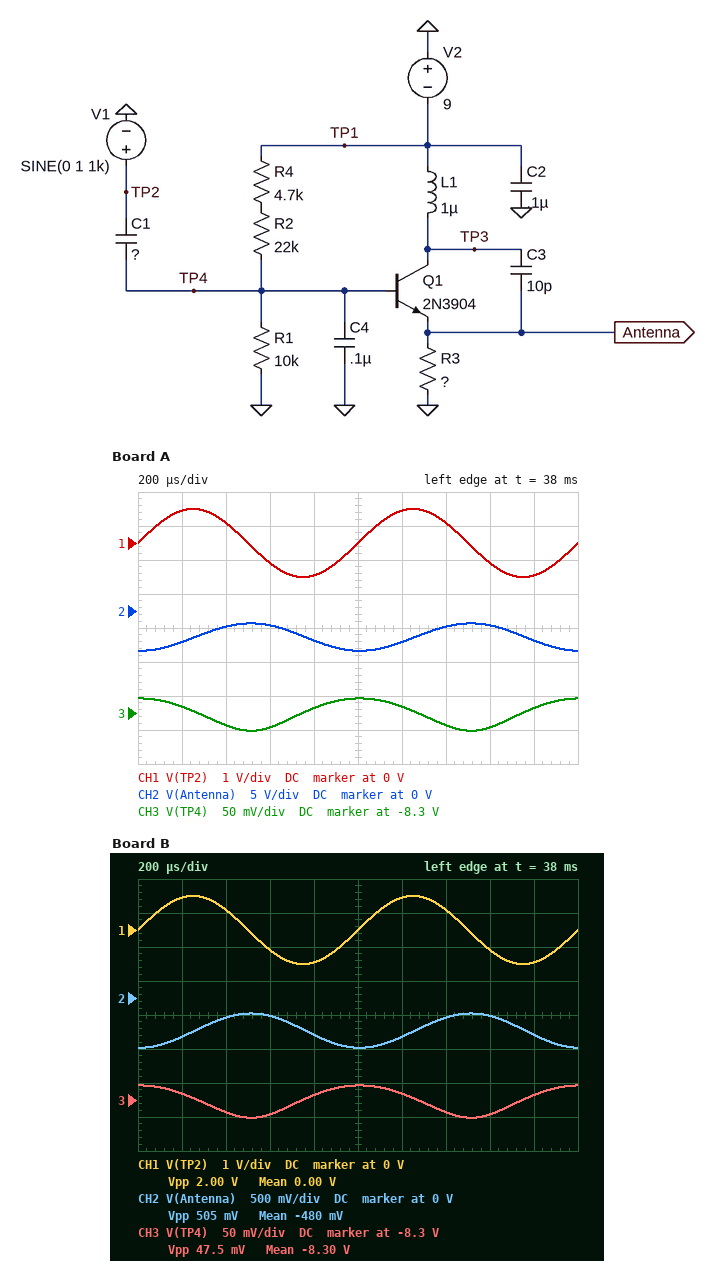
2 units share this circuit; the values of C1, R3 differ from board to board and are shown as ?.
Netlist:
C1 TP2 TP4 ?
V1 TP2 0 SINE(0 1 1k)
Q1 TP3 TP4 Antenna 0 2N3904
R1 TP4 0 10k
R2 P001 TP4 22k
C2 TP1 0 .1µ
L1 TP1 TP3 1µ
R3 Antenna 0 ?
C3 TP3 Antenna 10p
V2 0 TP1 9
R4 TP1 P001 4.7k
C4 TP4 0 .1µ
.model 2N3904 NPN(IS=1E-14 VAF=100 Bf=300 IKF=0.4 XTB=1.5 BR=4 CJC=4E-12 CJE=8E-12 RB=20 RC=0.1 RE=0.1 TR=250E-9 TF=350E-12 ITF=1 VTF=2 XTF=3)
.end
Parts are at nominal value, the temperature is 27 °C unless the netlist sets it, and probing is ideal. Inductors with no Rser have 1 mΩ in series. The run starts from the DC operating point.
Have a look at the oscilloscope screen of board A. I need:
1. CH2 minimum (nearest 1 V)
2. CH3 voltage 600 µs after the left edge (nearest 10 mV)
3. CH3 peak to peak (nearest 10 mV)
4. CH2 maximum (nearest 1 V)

-6 V
-8.32 V
50 mV
-2 V
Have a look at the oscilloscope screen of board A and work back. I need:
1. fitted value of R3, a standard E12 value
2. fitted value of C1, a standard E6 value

1.2 kΩ
68 nF
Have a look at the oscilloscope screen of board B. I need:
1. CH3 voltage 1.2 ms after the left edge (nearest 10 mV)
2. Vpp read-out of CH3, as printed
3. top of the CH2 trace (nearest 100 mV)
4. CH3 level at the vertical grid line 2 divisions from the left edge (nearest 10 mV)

-8.29 V
47.5 mV
-200 mV
-8.32 V
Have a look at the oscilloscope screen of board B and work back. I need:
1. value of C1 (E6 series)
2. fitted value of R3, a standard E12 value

68 nF
150 Ω
